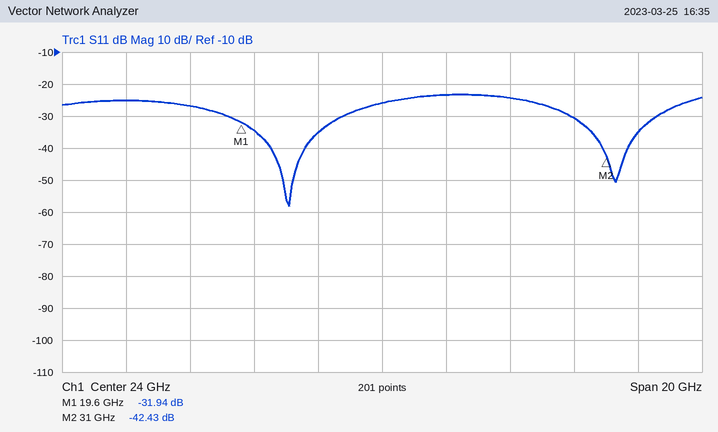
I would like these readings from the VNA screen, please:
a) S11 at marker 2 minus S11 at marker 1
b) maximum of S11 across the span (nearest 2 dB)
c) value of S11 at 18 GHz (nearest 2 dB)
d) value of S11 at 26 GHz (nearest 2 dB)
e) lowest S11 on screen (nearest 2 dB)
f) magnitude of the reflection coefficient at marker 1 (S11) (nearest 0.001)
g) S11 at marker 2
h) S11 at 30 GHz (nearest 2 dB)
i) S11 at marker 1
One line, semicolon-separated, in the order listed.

-10.49 dB; -24 dB; -26 dB; -24 dB; -58 dB; 0.025; -42.43 dB; -30 dB; -31.94 dB
